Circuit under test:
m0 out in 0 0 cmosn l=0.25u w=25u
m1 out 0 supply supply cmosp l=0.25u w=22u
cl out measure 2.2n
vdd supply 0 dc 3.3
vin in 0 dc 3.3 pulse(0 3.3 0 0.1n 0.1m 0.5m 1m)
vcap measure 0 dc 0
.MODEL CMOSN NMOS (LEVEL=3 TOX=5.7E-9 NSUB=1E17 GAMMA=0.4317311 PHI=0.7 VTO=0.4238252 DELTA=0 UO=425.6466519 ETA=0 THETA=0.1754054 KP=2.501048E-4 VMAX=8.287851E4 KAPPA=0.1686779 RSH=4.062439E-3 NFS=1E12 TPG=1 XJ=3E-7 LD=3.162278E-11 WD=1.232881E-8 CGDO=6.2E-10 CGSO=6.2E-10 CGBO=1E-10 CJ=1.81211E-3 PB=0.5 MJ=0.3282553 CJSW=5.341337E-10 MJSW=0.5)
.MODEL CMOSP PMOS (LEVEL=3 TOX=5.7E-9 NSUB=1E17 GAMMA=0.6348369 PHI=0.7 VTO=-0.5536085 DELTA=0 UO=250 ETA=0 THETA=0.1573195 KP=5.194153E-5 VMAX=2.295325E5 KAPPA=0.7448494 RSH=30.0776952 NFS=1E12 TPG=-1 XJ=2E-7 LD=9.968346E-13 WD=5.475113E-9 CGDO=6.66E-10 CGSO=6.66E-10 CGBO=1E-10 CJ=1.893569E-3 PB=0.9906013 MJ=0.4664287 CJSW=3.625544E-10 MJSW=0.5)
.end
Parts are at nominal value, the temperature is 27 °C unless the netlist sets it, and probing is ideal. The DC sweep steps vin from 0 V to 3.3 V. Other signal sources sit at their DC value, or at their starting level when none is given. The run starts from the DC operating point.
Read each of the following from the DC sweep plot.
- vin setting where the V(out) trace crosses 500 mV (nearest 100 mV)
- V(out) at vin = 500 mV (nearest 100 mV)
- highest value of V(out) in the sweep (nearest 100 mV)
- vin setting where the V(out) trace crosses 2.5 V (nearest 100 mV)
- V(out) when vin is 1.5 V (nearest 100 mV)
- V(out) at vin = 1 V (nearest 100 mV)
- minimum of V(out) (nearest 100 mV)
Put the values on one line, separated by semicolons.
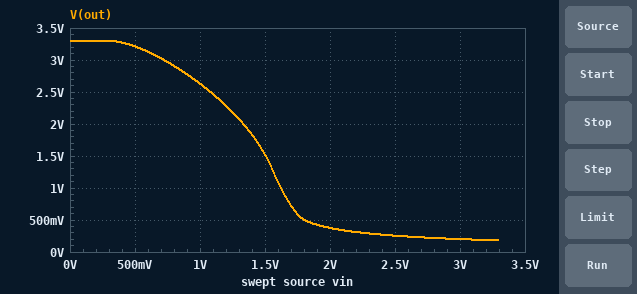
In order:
1.8 V; 3.2 V; 3.3 V; 1.1 V; 1.5 V; 2.6 V; 200 mV
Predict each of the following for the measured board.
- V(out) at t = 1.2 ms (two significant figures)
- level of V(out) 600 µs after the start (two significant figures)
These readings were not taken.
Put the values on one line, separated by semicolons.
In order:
180 mV; 3.3 V
